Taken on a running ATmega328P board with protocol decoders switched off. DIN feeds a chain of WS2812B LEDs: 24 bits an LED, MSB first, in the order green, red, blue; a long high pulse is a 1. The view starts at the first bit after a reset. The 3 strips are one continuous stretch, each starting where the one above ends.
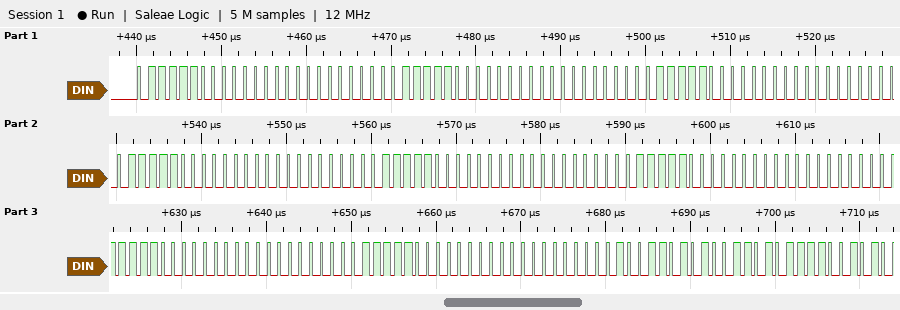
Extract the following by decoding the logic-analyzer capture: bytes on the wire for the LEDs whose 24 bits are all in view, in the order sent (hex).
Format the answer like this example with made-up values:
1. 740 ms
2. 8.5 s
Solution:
1. 7C 00 00 7C 00 00 7C 00 00 7C 00 00 7C 00 00 7C 00 00 7C 00 00 7C 00 00 4D 4D 79
